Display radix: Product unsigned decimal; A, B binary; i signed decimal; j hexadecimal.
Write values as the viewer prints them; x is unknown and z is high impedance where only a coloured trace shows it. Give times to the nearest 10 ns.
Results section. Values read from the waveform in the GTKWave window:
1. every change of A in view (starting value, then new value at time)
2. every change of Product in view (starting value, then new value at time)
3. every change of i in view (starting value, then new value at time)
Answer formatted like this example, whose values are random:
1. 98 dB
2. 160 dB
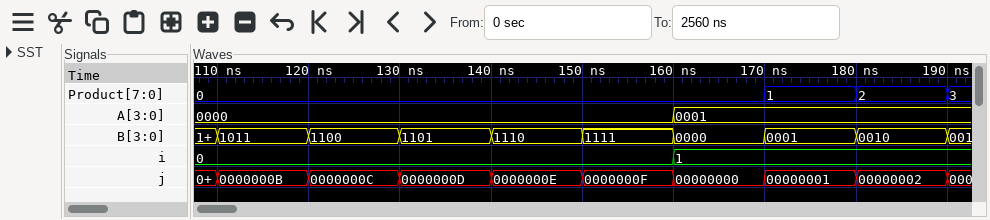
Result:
1. 0000, 0001 at 160 ns
2. 0, 1 at 170 ns, 2 at 180 ns, 3 at 190 ns
3. 0, 1 at 160 ns
